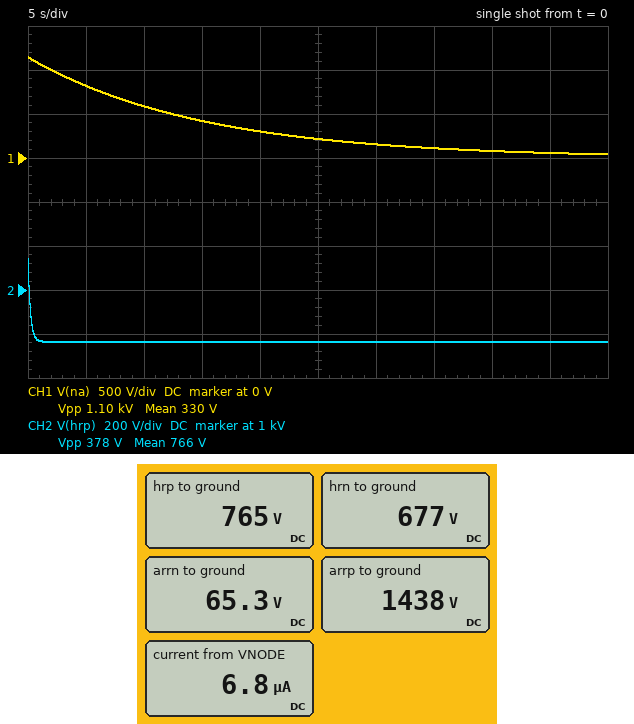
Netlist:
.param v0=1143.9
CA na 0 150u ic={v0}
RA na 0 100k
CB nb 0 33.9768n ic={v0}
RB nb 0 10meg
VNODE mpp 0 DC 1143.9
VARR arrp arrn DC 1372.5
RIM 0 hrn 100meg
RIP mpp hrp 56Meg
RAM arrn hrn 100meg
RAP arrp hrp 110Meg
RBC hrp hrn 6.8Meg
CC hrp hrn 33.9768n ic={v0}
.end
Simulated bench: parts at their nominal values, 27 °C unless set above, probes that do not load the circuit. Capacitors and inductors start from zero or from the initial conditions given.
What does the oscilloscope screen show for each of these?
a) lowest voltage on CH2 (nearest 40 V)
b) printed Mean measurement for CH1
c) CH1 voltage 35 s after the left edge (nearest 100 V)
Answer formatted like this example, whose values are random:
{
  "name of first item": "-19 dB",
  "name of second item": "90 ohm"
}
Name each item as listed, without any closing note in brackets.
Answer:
{
  "lowest voltage on CH2": "760 V",
  "printed Mean measurement for CH1": "330 V",
  "CH1 voltage 35 s after the left edge": "100 V"
}
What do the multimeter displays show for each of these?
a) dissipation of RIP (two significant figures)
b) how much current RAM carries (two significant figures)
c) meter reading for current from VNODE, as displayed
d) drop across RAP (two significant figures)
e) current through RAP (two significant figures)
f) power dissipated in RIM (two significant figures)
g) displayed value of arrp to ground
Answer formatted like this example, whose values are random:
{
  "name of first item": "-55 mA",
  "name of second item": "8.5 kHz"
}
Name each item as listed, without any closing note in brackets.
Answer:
{
  "dissipation of RIP": "2.6 mW",
  "how much current RAM carries": "6.1 µA",
  "meter reading for current from VNODE, as displayed": "6.8 µA",
  "drop across RAP": "670 V",
  "current through RAP": "6.1 µA",
  "power dissipated in RIM": "4.6 mW",
  "displayed value of arrp to ground": "1438 V"
}
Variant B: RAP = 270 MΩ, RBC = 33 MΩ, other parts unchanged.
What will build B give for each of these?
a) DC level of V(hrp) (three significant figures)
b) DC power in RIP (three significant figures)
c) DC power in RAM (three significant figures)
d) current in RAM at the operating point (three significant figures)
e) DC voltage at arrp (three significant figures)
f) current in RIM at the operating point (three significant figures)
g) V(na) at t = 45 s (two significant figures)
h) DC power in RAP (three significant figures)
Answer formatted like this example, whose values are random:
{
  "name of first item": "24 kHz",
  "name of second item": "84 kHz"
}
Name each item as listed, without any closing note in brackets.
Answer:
{
  "DC level of V(hrp)": "834 V",
  "DC power in RIP": "1.72 mW",
  "DC power in RAM": "872 µW",
  "current in RAM at the operating point": "2.95 µA",
  "DC voltage at arrp": "1.63 kV",
  "current in RIM at the operating point": "5.54 µA",
  "V(na) at t = 45 s": "57 V",
  "DC power in RAP": "2.35 mW"
}
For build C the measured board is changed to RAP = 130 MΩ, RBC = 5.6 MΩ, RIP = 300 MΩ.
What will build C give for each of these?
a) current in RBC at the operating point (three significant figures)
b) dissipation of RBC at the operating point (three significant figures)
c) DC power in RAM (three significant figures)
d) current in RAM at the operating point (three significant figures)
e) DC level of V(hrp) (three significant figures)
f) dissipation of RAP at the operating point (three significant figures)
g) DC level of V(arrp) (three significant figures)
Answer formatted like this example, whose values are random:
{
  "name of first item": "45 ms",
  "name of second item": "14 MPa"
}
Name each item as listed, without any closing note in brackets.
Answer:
{
  "current in RBC at the operating point": "8.50 µA",
  "dissipation of RBC at the operating point": "405 µW",
  "DC power in RAM": "3.32 mW",
  "current in RAM at the operating point": "5.76 µA",
  "DC level of V(hrp)": "322 V",
  "dissipation of RAP at the operating point": "4.31 mW",
  "DC level of V(arrp)": "1.07 kV"
}
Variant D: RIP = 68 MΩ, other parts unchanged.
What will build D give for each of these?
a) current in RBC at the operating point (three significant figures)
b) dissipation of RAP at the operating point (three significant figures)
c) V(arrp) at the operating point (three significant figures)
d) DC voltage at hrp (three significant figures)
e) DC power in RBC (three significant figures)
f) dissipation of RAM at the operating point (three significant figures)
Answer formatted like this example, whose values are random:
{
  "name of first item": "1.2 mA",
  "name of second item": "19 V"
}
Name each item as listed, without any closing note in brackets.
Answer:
{
  "current in RBC at the operating point": "12.4 µA",
  "dissipation of RAP at the operating point": "4.14 mW",
  "V(arrp) at the operating point": "1.39 kV",
  "DC voltage at hrp": "715 V",
  "DC power in RBC": "1.05 mW",
  "dissipation of RAM at the operating point": "3.76 mW"
}
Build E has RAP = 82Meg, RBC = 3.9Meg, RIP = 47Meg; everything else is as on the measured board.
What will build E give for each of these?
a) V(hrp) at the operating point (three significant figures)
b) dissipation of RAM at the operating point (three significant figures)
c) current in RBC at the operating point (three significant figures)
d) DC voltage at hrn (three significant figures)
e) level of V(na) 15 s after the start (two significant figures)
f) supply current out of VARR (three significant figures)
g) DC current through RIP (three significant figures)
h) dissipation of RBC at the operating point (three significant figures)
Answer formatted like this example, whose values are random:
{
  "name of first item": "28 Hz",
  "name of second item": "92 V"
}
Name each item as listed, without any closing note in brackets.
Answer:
{
  "V(hrp) at the operating point": "796 V",
  "dissipation of RAM at the operating point": "5.22 mW",
  "current in RBC at the operating point": "14.6 µA",
  "DC voltage at hrn": "739 V",
  "level of V(na) 15 s after the start": "420 V",
  "supply current out of VARR": "7.23 µA",
  "DC current through RIP": "7.39 µA",
  "dissipation of RBC at the operating point": "834 µW"
}
